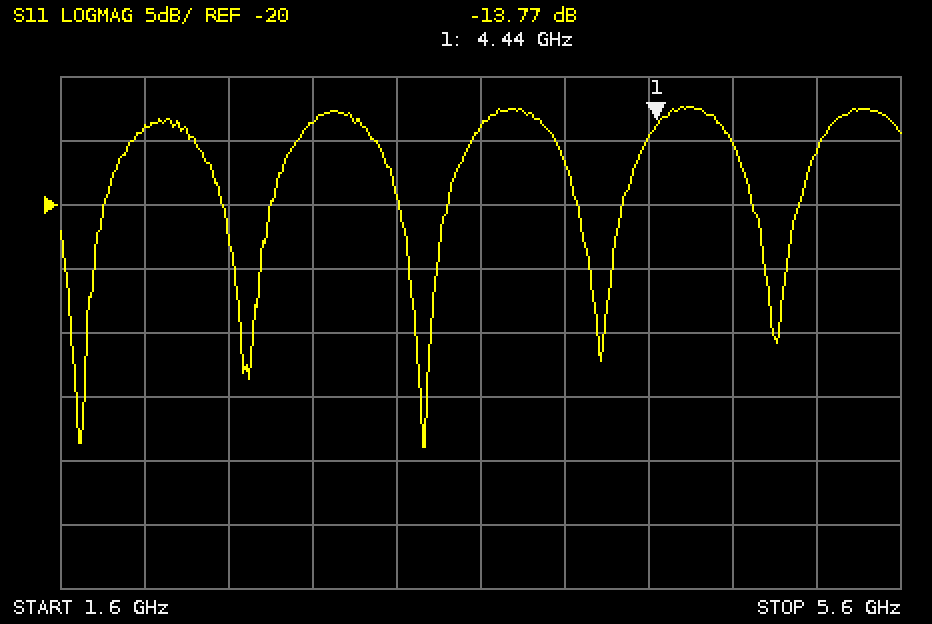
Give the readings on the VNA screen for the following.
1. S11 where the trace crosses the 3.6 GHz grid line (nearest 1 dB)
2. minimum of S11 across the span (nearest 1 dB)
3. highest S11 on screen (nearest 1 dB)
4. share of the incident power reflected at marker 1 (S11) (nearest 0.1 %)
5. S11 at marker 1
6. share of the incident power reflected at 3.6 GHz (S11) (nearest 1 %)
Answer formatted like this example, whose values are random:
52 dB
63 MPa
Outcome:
-14 dB
-39 dB
-12 dB
4.2 %
-13.77 dB
4 %
